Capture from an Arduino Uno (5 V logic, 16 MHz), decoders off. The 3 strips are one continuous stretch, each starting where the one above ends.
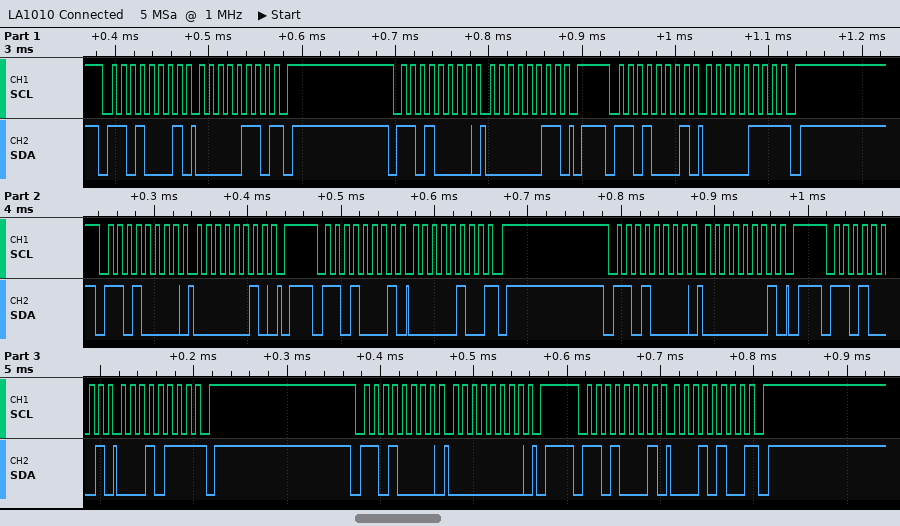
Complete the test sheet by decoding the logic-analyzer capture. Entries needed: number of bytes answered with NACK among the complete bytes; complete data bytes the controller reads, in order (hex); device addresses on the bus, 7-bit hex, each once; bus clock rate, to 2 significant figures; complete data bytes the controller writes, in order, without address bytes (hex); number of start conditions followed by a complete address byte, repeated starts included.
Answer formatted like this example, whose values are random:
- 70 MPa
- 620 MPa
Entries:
- 5
- 06 07 04 17 14
- 0x68
- 100 kHz
- 03 02 01 00
- 9
